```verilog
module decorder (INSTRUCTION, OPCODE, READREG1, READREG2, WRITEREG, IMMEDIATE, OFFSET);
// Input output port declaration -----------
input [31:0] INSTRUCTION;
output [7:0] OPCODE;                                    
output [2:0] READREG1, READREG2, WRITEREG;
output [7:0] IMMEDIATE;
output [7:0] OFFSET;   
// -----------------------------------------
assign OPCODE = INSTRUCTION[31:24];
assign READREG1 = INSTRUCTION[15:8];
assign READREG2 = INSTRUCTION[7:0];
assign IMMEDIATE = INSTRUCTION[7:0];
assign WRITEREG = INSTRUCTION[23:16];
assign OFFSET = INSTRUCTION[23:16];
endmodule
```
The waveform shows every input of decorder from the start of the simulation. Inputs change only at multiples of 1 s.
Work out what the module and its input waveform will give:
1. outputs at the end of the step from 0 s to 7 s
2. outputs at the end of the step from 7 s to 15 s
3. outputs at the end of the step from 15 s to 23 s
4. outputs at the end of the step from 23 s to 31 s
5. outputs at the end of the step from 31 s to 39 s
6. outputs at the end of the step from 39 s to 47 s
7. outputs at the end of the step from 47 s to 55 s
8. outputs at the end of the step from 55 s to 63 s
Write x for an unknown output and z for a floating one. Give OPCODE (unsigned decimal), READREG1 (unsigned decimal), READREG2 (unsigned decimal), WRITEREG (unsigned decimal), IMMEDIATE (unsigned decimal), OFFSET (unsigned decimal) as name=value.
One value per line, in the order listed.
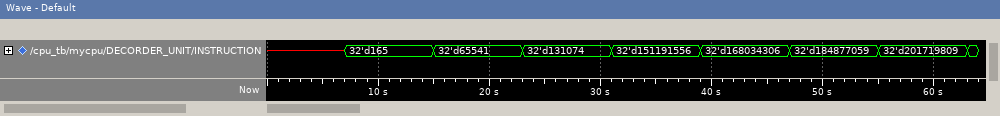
OPCODE=x, READREG1=x, READREG2=x, WRITEREG=x, IMMEDIATE=x, OFFSET=x
OPCODE=0, READREG1=0, READREG2=5, WRITEREG=0, IMMEDIATE=165, OFFSET=0
OPCODE=0, READREG1=0, READREG2=5, WRITEREG=1, IMMEDIATE=5, OFFSET=1
OPCODE=0, READREG1=0, READREG2=2, WRITEREG=2, IMMEDIATE=2, OFFSET=2
OPCODE=9, READREG1=0, READREG2=4, WRITEREG=3, IMMEDIATE=4, OFFSET=3
OPCODE=10, READREG1=0, READREG2=2, WRITEREG=4, IMMEDIATE=2, OFFSET=4
OPCODE=11, READREG1=0, READREG2=3, WRITEREG=5, IMMEDIATE=3, OFFSET=5
OPCODE=12, READREG1=0, READREG2=1, WRITEREG=6, IMMEDIATE=1, OFFSET=6
